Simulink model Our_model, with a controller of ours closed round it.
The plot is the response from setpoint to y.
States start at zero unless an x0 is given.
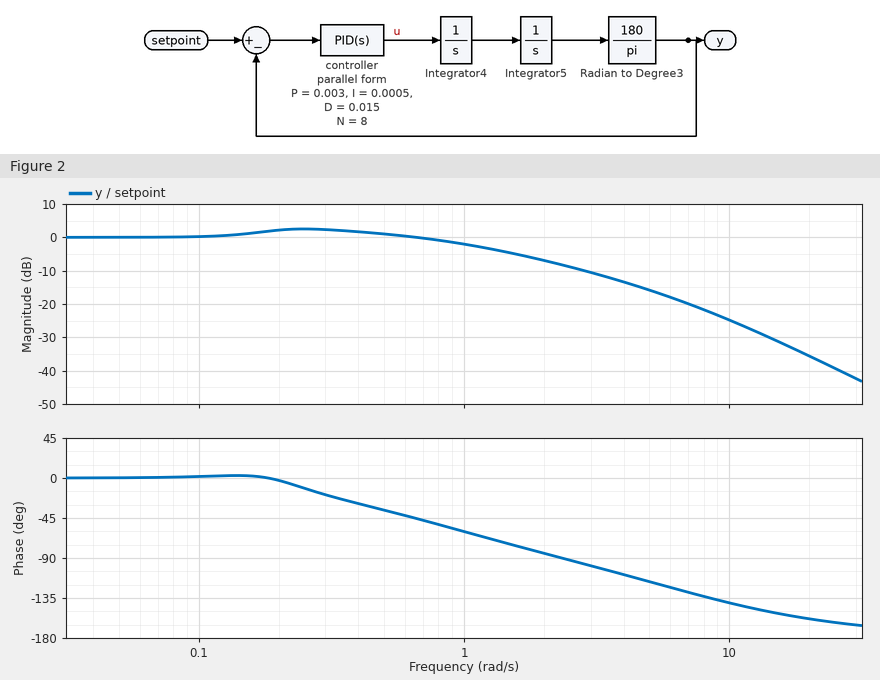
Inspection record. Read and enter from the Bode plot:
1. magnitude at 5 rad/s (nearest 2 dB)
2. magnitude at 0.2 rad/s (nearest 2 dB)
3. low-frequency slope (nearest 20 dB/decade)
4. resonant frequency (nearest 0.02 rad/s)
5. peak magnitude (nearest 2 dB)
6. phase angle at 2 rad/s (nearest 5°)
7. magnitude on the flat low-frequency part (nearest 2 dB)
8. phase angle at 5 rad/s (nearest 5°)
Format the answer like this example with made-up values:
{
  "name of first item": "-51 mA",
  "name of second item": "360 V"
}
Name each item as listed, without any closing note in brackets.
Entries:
{
  "magnitude at 5 rad/s": "-16 dB",
  "magnitude at 0.2 rad/s": "2 dB",
  "low-frequency slope": "0 dB/decade",
  "resonant frequency": "0.26 rad/s",
  "peak magnitude": "2 dB",
  "phase angle at 2 rad/s": "-85°",
  "magnitude on the flat low-frequency part": "0 dB",
  "phase angle at 5 rad/s": "-115°"
}
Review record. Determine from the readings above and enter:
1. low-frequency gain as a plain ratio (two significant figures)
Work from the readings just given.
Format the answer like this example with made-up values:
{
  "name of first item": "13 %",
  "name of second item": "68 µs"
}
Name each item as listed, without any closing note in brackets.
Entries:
{
  "low-frequency gain as a plain ratio": "1.0"
}
